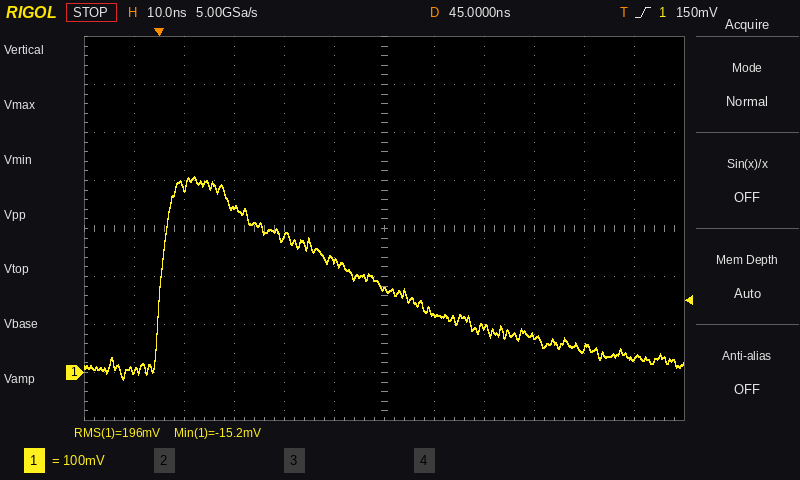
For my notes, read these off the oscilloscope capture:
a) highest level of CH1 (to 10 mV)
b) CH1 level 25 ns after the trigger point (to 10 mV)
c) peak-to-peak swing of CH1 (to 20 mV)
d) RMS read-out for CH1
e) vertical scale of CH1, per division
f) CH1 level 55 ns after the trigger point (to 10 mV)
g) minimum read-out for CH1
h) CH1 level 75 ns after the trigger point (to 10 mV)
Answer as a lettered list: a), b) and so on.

a) 410 mV
b) 280 mV
c) 420 mV
d) 196 mV
e) 100 mV
f) 120 mV
g) -15.2 mV
h) 80 mV
